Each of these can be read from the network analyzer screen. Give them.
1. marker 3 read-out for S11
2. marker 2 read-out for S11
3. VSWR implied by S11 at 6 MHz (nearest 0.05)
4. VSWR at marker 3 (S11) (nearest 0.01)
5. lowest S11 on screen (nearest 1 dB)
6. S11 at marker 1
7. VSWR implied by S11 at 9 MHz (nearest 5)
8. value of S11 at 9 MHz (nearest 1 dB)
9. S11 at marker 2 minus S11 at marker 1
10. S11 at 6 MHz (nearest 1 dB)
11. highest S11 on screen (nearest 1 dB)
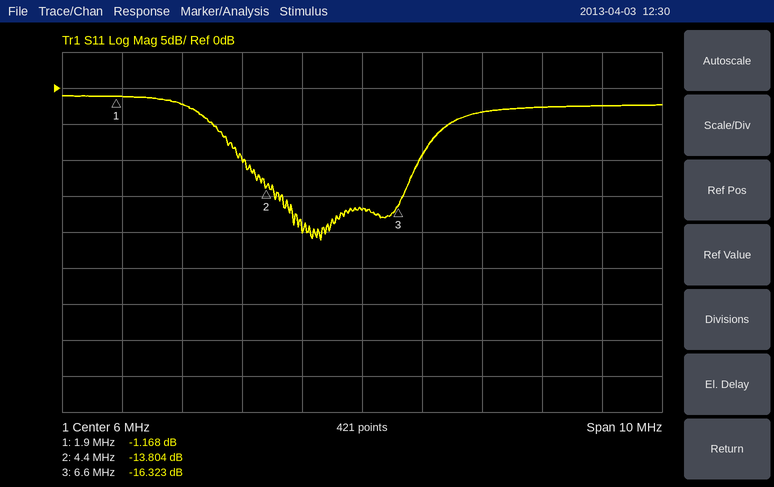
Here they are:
-16.323 dB
-13.804 dB
1.35
1.36
-21 dB
-1.168 dB
5
-3 dB
-12.636 dB
-17 dB
-1 dB
